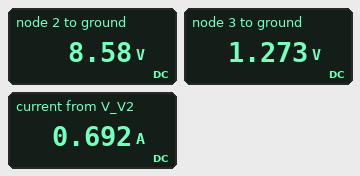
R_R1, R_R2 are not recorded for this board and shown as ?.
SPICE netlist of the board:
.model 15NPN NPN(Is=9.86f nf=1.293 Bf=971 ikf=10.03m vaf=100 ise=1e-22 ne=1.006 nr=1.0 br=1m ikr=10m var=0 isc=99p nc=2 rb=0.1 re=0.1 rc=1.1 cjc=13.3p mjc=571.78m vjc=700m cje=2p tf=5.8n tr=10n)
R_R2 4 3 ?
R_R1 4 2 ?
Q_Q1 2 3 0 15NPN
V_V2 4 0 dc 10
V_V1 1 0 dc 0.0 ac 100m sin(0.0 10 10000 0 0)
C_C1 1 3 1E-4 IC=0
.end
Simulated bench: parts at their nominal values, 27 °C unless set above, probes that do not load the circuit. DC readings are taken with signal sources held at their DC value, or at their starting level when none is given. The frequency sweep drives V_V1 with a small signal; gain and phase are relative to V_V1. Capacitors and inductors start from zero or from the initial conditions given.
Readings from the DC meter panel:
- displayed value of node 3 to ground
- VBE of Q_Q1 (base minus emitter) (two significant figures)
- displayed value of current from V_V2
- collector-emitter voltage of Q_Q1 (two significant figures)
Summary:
1.273 V
1.3 V
0.692 A
8.6 V
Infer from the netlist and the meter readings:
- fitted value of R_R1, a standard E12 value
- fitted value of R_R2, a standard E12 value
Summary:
2.2 Ω
180 Ω
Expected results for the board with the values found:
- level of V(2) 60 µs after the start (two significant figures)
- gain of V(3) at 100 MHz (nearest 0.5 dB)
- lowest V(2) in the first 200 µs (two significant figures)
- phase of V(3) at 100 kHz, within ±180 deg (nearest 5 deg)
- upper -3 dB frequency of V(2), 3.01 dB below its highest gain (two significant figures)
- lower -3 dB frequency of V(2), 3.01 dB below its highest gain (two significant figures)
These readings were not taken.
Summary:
10 V
0 dB
4.1 V
0 deg
33 MHz
1.1 kHz
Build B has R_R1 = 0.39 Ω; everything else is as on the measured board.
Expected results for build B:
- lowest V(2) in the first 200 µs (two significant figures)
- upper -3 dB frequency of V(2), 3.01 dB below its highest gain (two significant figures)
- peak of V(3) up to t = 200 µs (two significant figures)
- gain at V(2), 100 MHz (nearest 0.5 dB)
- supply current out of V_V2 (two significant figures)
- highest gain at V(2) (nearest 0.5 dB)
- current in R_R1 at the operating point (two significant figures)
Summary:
7.9 V
32 MHz
6.7 V
-6.0 dB
700 mA
4.5 dB
650 mA
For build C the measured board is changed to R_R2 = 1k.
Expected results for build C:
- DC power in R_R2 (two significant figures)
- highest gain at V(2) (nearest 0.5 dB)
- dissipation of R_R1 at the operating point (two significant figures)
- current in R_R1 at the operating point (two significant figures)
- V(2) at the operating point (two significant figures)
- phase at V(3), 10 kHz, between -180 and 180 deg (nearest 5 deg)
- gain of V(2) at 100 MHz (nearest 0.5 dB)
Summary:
78 mW
16.0 dB
180 mW
290 mA
9.4 V
0 deg
8.5 dB
